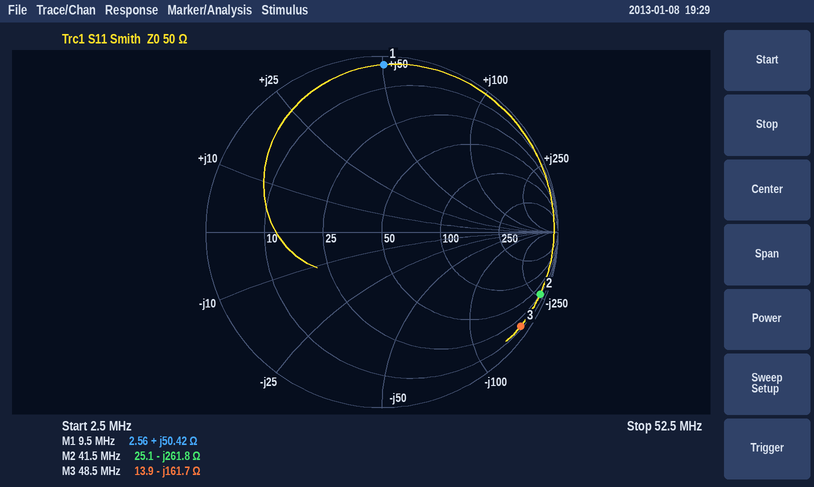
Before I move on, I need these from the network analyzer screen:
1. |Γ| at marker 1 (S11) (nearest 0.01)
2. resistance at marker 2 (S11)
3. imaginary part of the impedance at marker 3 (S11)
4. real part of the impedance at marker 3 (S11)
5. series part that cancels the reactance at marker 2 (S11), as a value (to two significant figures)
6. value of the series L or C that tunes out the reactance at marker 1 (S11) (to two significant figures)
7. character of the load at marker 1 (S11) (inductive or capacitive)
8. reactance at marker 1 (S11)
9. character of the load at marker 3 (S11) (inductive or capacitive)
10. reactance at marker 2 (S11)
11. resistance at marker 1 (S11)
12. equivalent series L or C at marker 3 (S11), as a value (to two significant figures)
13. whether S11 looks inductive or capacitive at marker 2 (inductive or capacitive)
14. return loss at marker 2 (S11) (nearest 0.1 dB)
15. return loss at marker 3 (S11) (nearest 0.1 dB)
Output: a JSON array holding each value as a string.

["0.95", "25.1 Ω", "-161.7 Ω", "13.9 Ω", "1.0 µH", "330 pF", "inductive", "+50.42 Ω", "capacitive", "-261.8 Ω", "2.56 Ω", "20 pF", "capacitive", "0.3 dB", "0.4 dB"]
